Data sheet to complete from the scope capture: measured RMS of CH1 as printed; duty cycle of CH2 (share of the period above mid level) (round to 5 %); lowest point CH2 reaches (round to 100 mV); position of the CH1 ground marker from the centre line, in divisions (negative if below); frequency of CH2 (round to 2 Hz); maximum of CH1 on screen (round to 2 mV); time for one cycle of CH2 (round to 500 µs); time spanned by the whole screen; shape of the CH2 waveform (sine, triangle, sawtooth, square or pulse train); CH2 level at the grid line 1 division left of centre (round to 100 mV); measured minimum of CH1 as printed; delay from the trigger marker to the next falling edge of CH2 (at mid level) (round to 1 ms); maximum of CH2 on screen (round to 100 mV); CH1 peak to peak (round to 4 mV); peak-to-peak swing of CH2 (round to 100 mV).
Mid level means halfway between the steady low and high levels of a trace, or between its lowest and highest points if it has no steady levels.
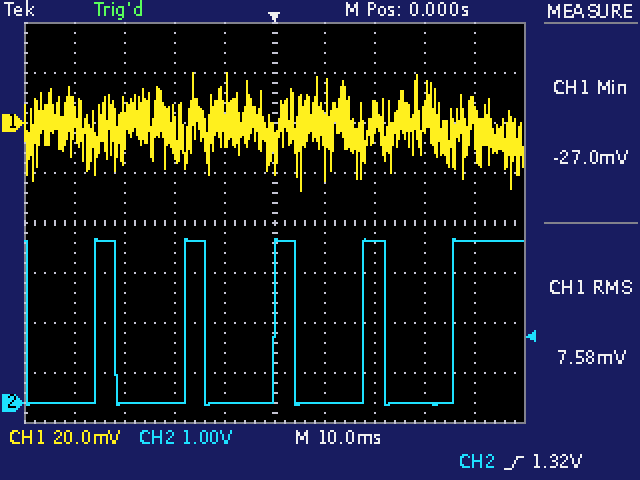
7.58 mV
25 %
0.0 V
+2.0 div
56 Hz
20 mV
18.0 ms
100 ms
pulse train
0.0 V
-27.0 mV
4 ms
3.3 V
48 mV
3.3 V
